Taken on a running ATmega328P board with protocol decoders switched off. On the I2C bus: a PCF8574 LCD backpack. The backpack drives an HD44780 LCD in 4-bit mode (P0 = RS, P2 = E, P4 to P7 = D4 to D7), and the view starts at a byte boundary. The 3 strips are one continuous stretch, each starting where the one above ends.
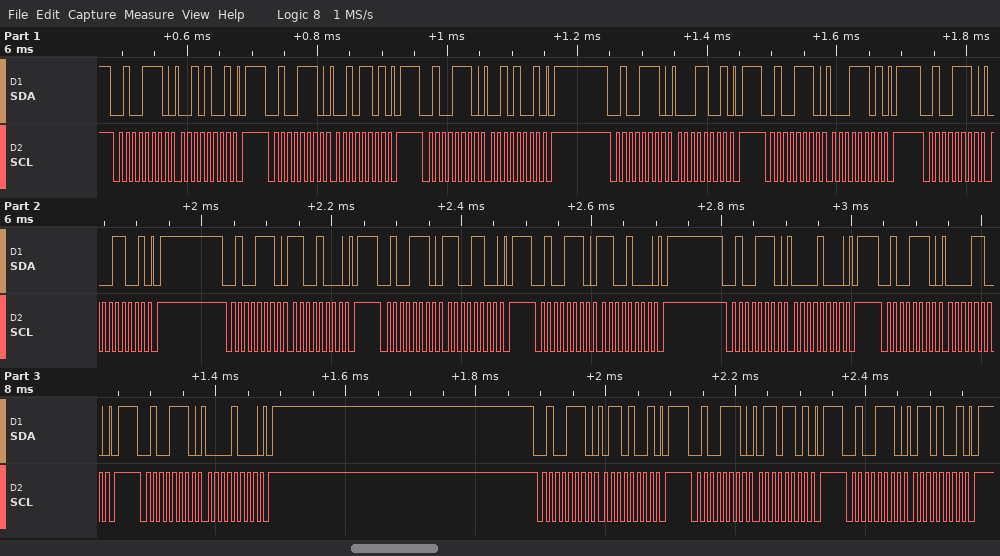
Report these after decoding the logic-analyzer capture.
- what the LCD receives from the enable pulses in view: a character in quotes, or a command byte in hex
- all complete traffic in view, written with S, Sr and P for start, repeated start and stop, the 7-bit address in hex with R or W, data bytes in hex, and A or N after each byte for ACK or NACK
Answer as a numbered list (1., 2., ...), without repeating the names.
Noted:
1. '!' 0xC0
2. S 27W A 29 A P S 27W A 2D A P S 27W A 29 A P S 27W A 19 A P S 27W A 1D A P S 27W A 19 A P S 27W A C8 A P S 27W A CC A P S 27W A C8 A P S 27W A 08 A P S 27W A 0C A P S 27W A 08 A P S 27W A 69 A P S 27W A 6D A P S 27W A 69 A P
